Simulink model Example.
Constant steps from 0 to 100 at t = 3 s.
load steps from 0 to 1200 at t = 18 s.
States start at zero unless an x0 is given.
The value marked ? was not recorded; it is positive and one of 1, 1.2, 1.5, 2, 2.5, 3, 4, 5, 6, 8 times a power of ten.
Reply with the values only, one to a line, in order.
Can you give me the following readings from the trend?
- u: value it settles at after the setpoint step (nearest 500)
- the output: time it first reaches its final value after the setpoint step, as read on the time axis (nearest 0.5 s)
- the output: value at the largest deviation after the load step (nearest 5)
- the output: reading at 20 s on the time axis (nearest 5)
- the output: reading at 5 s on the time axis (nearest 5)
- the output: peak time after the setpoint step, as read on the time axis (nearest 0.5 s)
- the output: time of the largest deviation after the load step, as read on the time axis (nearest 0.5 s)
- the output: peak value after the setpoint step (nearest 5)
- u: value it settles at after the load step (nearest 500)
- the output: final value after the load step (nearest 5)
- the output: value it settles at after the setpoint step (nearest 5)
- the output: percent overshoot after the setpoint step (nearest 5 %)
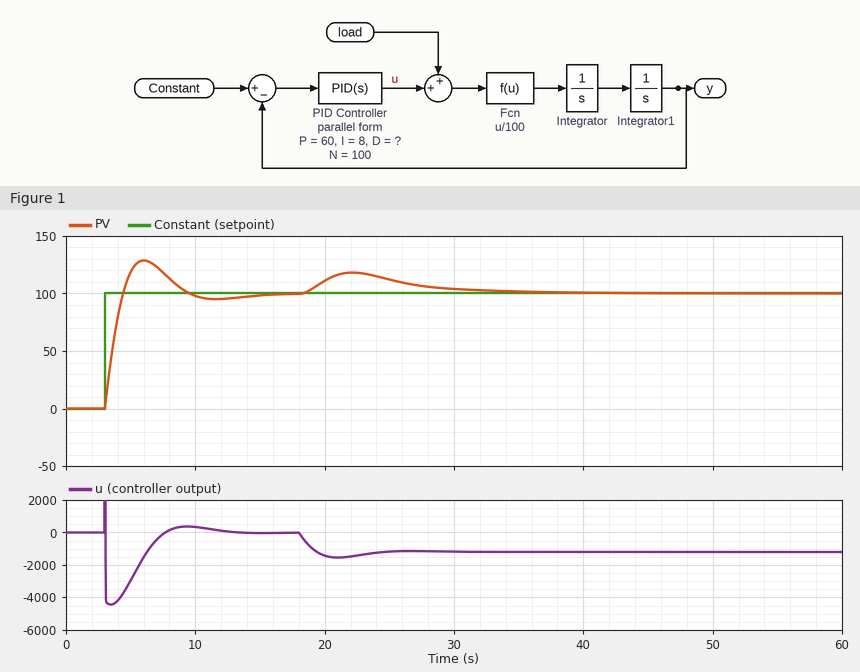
0
4.5 s
120
110
120
6.0 s
22.0 s
130
-1000
100
100
30 %
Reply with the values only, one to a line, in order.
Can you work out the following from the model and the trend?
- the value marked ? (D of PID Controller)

100
